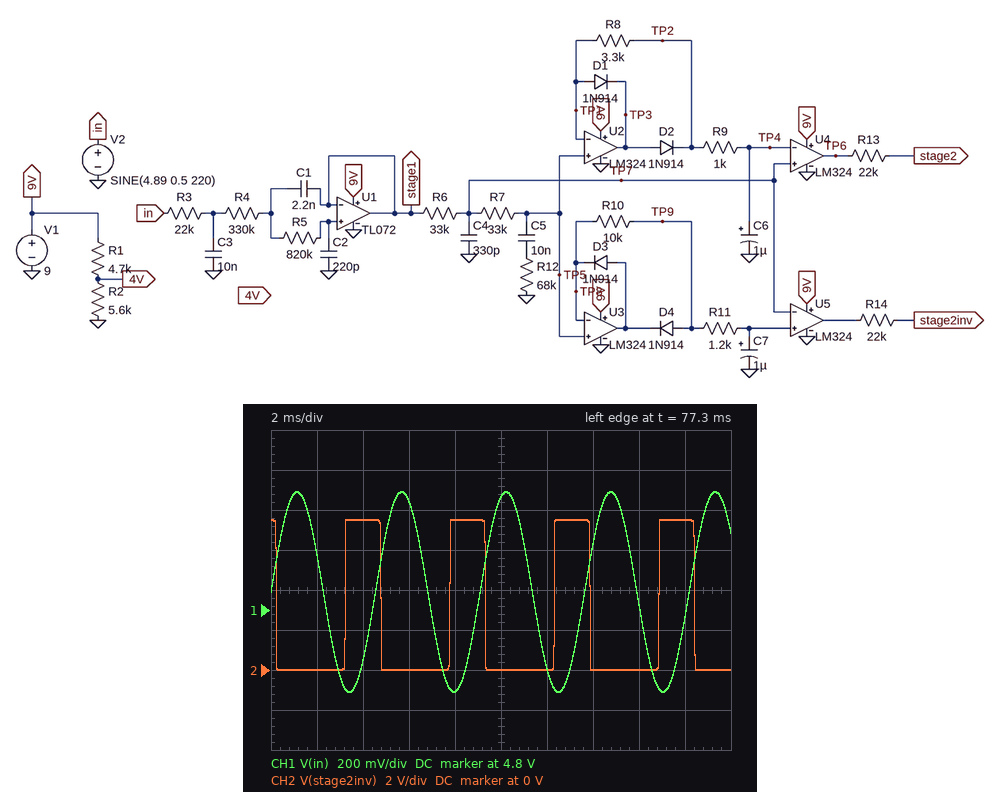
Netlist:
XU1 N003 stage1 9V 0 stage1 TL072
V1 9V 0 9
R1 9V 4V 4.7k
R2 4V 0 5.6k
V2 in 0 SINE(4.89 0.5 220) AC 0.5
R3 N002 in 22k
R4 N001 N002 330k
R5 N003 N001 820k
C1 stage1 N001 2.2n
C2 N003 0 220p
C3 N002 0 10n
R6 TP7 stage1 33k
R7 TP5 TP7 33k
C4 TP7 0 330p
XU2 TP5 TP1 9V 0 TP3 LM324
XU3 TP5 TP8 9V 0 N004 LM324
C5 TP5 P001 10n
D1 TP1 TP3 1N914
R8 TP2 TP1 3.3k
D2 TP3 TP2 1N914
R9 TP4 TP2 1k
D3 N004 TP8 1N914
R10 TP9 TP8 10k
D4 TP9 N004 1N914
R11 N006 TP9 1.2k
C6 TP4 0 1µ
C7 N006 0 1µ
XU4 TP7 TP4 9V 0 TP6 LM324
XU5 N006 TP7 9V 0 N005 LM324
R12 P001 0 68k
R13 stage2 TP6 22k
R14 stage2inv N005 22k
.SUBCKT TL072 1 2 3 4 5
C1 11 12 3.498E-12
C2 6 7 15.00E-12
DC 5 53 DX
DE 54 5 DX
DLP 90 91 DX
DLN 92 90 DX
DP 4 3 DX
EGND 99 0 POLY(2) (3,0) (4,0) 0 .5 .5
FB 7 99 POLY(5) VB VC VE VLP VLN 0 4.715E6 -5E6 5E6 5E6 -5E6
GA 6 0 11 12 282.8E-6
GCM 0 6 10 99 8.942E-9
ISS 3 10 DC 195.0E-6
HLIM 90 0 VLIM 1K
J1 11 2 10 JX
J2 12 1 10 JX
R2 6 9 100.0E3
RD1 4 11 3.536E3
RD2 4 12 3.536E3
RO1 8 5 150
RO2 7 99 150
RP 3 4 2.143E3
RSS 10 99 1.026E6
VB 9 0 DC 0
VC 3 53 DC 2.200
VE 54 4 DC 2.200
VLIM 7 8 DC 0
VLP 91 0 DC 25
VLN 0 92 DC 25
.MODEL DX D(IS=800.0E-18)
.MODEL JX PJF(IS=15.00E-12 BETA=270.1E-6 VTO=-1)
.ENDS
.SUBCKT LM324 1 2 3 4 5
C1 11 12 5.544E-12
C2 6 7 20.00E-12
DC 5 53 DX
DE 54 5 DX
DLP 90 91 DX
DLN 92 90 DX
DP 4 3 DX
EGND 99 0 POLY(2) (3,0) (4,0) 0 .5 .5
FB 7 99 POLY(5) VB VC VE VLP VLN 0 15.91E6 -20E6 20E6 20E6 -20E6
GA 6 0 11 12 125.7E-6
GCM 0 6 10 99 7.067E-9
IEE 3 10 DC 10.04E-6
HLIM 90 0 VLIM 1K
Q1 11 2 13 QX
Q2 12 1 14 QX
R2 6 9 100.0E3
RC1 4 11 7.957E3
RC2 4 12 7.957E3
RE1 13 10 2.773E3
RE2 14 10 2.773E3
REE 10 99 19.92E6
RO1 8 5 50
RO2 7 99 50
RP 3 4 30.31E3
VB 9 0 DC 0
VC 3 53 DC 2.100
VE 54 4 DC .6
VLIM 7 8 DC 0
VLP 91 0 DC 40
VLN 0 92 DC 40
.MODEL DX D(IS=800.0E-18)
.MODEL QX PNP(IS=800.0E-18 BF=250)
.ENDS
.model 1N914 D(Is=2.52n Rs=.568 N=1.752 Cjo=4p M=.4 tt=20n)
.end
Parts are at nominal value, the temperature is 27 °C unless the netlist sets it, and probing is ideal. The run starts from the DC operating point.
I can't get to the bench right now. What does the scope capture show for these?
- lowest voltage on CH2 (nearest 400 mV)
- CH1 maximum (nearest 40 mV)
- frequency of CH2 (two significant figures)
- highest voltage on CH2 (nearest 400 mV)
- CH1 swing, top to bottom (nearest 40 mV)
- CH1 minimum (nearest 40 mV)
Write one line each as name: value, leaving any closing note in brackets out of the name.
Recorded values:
lowest voltage on CH2: 0 V
CH1 maximum: 5.40 V
frequency of CH2: 220 Hz
highest voltage on CH2: 7.6 V
CH1 swing, top to bottom: 1.00 V
CH1 minimum: 4.40 V
